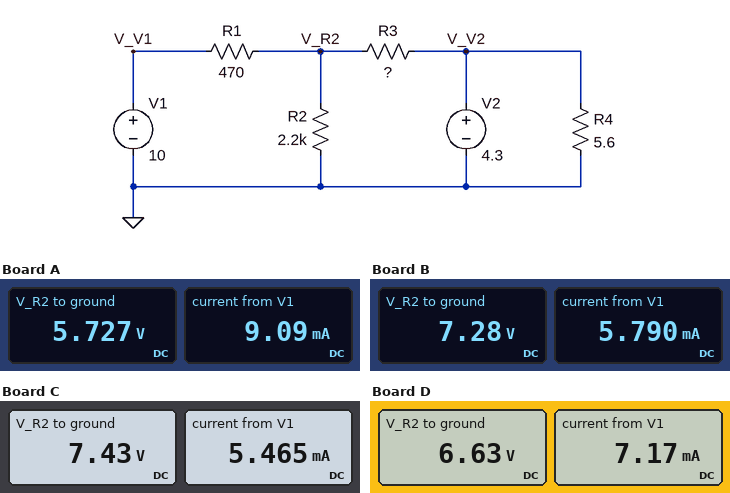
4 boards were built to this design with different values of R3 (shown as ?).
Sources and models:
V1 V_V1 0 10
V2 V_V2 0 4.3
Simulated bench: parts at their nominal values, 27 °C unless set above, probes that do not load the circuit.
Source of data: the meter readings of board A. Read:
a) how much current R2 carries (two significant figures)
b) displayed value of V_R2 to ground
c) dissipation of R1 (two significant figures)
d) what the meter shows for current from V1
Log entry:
2.6 mA
5.727 V
39 mW
9.09 mA
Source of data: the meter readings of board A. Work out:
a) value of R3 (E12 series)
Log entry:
220 Ω
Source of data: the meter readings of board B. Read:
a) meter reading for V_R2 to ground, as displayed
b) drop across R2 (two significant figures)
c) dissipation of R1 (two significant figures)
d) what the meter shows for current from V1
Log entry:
7.28 V
7.3 V
16 mW
5.790 mA
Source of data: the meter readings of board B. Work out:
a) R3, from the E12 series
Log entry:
1.2 kΩ
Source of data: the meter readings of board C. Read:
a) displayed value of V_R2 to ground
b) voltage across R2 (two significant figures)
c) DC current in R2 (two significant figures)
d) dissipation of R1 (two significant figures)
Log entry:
7.43 V
7.4 V
3.4 mA
14 mW
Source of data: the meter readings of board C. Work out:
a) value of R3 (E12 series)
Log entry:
1.5 kΩ
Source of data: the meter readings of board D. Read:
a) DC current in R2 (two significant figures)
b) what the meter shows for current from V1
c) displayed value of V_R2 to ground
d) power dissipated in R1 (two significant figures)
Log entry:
3.0 mA
7.17 mA
6.63 V
24 mW
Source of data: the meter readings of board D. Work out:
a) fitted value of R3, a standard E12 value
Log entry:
560 Ω
